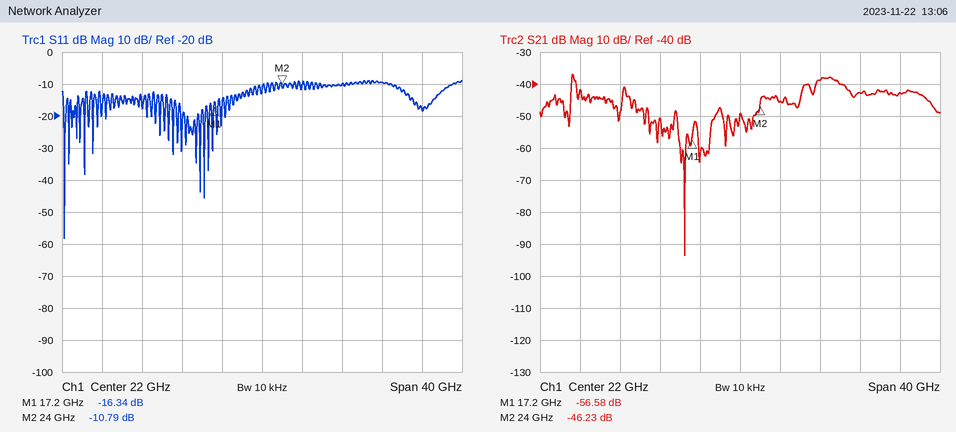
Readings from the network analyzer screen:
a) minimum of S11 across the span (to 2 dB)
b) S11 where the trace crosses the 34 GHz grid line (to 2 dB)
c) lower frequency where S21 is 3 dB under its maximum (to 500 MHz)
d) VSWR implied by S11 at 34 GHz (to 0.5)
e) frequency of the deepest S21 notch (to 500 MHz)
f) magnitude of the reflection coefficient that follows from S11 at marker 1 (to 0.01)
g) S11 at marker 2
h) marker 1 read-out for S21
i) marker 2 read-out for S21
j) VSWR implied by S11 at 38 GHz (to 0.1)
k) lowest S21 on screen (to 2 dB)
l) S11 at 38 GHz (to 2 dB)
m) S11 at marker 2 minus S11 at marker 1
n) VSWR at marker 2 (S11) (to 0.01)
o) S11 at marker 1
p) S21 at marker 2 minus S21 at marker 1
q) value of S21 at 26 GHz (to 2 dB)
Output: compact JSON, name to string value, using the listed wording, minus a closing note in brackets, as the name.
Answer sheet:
{"minimum of S11 across the span": "-58 dB", "S11 where the trace crosses the 34 GHz grid line": "-10 dB", "lower frequency where S21 is 3 dB under its maximum": "5.0 GHz", "VSWR implied by S11 at 34 GHz": "2.0", "frequency of the deepest S21 notch": "16.5 GHz", "magnitude of the reflection coefficient that follows from S11 at marker 1": "0.15", "S11 at marker 2": "-10.79 dB", "marker 1 read-out for S21": "-56.58 dB", "marker 2 read-out for S21": "-46.23 dB", "VSWR implied by S11 at 38 GHz": "1.3", "lowest S21 on screen": "-94 dB", "S11 at 38 GHz": "-18 dB", "S11 at marker 2 minus S11 at marker 1": "5.55 dB", "VSWR at marker 2 (S11)": "1.81", "S11 at marker 1": "-16.34 dB", "S21 at marker 2 minus S21 at marker 1": "10.35 dB", "value of S21 at 26 GHz": "-46 dB"}
